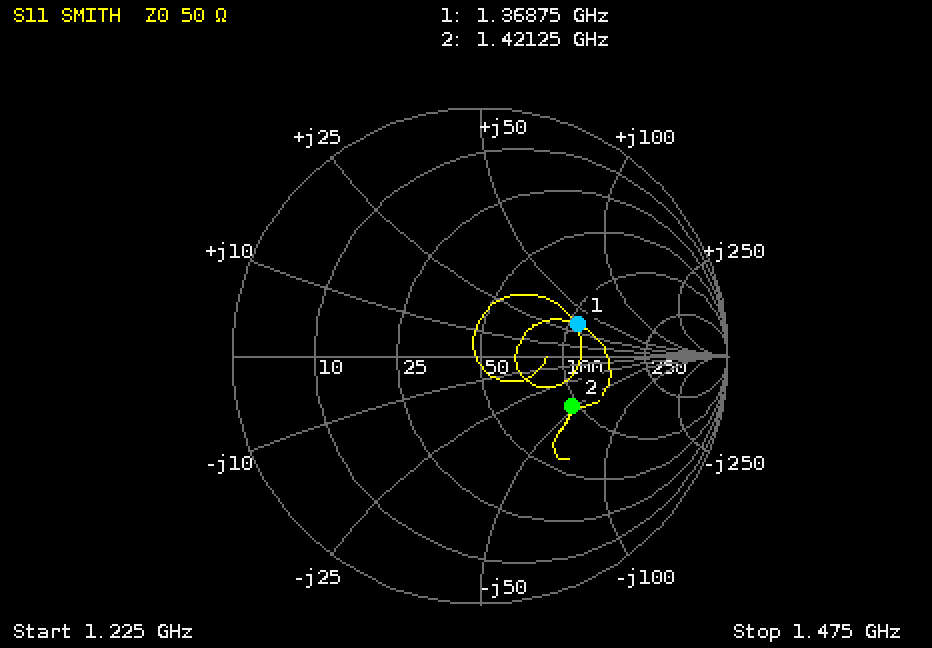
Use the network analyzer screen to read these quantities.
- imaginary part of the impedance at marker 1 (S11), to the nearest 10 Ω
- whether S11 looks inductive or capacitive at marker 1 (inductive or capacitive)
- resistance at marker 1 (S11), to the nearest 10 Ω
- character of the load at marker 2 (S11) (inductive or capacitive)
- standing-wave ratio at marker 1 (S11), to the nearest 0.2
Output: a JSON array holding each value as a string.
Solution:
["+30 Ω", "inductive", "110 Ω", "capacitive", "2.4"]
